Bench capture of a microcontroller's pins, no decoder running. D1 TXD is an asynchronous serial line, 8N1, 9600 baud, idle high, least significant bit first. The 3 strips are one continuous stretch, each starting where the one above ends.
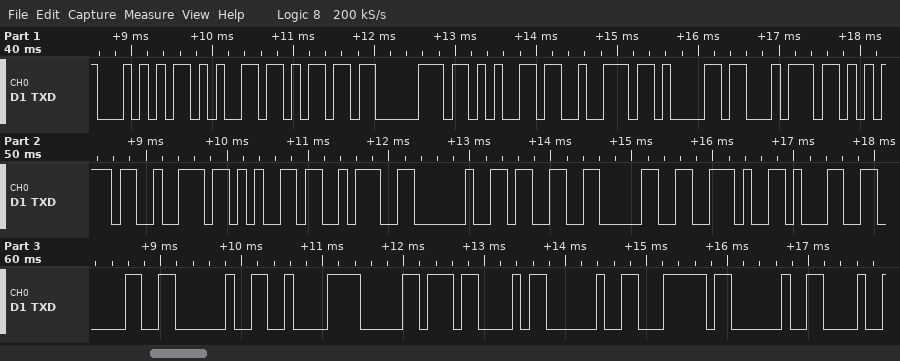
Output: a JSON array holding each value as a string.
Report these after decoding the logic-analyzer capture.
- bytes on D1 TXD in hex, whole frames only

["0x54 0x65 0x6D 0x70 0x65 0x72 0x61 0x74 0x75 0x72 0x65 0x3A 0x20 0x33 0x30 0x2E 0x31 0x30 0x20 0xC2 0xB0 0x43 0x20 0x7C 0x20"]
